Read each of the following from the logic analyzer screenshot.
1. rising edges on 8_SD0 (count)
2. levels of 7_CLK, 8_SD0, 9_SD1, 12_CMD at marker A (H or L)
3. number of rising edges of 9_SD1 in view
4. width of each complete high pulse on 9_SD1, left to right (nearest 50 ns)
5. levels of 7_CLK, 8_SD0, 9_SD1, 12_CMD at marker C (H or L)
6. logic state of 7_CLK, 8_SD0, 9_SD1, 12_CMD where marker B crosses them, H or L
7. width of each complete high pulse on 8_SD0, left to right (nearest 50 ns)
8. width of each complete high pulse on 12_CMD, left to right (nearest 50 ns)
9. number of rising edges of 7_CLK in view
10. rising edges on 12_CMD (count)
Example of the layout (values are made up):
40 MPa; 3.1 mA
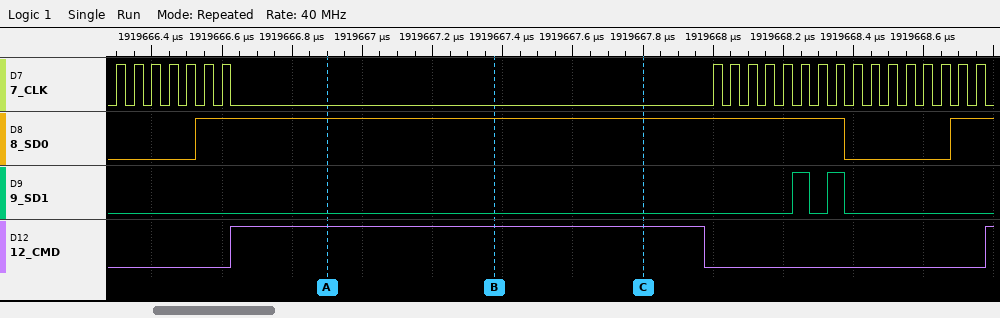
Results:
2; 7_CLK=L, 8_SD0=H, 9_SD1=L, 12_CMD=H; 2; 50 ns, 50 ns; 7_CLK=L, 8_SD0=H, 9_SD1=L, 12_CMD=H; 7_CLK=L, 8_SD0=H, 9_SD1=L, 12_CMD=H; 1850 ns; 1350 ns; 23; 2
